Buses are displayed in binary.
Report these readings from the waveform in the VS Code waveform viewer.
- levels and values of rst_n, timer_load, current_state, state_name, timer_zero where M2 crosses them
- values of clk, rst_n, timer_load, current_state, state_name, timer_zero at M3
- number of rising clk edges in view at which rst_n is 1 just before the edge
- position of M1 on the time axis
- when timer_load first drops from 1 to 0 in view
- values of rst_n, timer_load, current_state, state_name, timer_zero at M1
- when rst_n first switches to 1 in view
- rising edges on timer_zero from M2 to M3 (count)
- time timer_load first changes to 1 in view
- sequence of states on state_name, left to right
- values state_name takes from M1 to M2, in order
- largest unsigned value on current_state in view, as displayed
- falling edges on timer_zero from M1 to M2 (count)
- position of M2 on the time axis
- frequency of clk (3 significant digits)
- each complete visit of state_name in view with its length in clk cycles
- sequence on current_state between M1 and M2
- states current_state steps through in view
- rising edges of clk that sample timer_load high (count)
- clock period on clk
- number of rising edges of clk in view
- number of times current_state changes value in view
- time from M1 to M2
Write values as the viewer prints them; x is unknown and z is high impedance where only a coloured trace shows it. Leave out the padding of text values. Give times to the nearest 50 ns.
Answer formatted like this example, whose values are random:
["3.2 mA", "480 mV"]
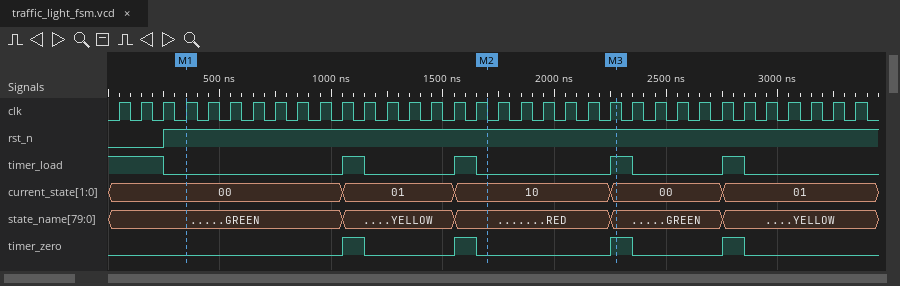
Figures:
["rst_n=1, timer_load=0, current_state=10, state_name=RED, timer_zero=0", "clk=1, rst_n=1, timer_load=1, current_state=00, state_name=GREEN, timer_zero=1", "31", "350 ns", "250 ns", "rst_n=1, timer_load=0, current_state=00, state_name=GREEN, timer_zero=0", "250 ns", "1", "1050 ns", "GREEN, YELLOW, RED, GREEN, YELLOW", "GREEN, YELLOW, RED", "10", "2", "1700 ns", "10.0 MHz", "YELLOW: 5, RED: 7, GREEN: 5", "00, 01, 10", "00, 01, 10, 00, 01", "7", "100 ns", "34", "4", "1350 ns"]
